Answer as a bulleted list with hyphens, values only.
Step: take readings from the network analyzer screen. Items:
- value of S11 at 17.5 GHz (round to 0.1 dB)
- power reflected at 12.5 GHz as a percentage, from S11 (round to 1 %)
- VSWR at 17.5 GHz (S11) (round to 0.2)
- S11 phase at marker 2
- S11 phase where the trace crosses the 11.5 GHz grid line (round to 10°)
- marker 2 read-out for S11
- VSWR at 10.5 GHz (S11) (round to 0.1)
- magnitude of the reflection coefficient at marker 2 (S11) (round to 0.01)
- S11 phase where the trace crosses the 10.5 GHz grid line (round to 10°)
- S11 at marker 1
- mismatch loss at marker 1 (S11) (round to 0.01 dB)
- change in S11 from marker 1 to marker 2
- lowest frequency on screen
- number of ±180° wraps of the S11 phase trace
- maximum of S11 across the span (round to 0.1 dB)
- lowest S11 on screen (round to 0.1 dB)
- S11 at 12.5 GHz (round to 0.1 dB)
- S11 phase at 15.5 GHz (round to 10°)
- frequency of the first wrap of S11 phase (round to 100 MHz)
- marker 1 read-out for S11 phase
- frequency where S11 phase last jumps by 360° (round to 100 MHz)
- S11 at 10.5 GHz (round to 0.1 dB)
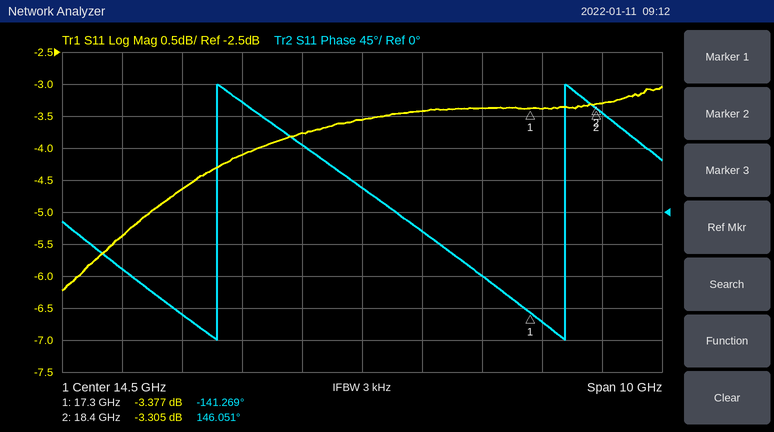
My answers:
- -3.4 dB
- 39 %
- 5.2
- 146.051°
- -140°
- -3.305 dB
- 3.3
- 0.68
- -80°
- -3.377 dB
- 2.67 dB
- 0.072 dB
- 9.5 GHz
- 2
- -3.0 dB
- -6.2 dB
- -4.1 dB
- -30°
- 12.1 GHz
- -141.269°
- 17.9 GHz
- -5.4 dB
